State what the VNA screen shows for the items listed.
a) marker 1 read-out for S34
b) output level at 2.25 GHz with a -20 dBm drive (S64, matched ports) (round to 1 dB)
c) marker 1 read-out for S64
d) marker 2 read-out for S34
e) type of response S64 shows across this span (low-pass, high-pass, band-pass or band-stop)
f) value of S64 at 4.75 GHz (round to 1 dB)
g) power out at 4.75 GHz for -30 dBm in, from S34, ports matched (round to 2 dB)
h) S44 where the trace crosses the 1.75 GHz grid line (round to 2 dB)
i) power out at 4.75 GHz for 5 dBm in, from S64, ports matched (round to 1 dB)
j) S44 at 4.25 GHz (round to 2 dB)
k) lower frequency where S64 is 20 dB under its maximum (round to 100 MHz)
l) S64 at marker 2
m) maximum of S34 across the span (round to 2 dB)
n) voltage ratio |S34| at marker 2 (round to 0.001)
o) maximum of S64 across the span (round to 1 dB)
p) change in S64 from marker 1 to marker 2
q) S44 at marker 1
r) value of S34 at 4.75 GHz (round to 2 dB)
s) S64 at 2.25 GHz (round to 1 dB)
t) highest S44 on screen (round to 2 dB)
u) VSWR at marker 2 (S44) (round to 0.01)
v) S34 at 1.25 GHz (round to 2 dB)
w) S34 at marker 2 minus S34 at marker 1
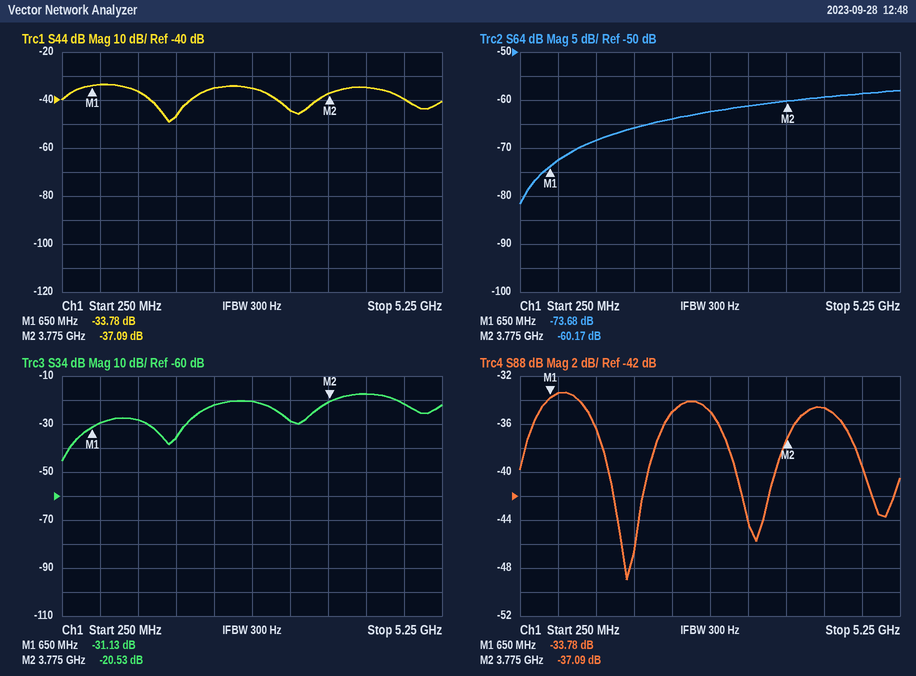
-31.13 dB
-84 dBm
-73.68 dB
-20.53 dB
high-pass
-59 dB
-52 dBm
-46 dB
-54 dBm
-34 dB
400 MHz
-60.17 dB
-18 dB
0.094
-58 dB
13.51 dB
-33.78 dB
-22 dB
-64 dB
-34 dB
1.03
-28 dB
10.60 dB
